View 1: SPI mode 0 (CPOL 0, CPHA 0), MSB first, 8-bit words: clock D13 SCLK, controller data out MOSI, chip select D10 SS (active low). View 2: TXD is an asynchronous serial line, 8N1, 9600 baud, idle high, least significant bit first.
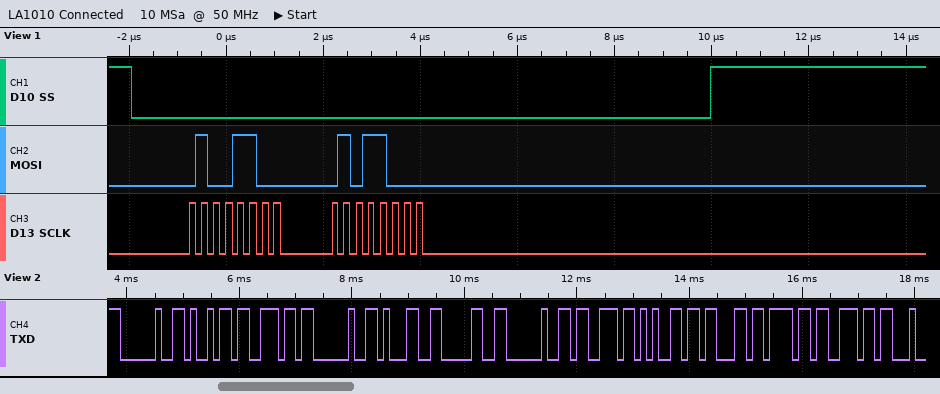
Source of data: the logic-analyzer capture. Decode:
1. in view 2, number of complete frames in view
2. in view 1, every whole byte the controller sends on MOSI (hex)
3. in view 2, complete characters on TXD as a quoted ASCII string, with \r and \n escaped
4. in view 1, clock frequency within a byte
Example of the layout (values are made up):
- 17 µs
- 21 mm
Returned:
- 12
- 0x4C 0x58
- " in 10 secon"
- 4 MHz
